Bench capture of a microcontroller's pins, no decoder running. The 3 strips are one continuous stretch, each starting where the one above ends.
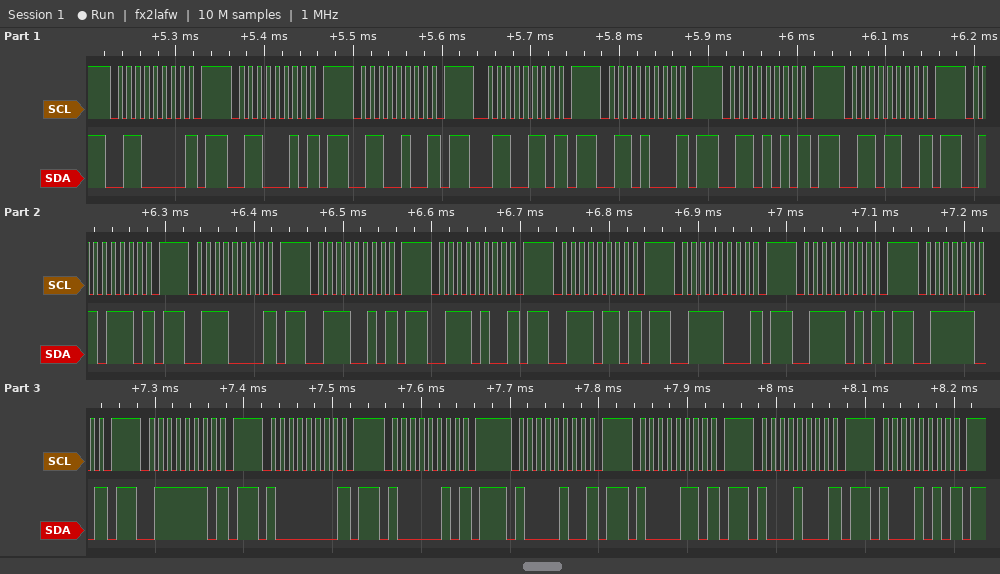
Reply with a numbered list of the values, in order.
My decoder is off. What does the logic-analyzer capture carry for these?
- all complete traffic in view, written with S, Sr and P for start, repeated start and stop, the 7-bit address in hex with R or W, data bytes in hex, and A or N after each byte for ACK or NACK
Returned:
1. S 30W N P S 31W N P S 32W N P S 33W N P S 34W N P S 35W N P S 36W N P S 37W N P S 38W N P S 39W N P S 3AW N P S 3BW N P S 3CW N P S 3DW N P S 3EW N P S 3FW N P S 40W N P S 41W N P S 42W N P S 43W N P S 44W N P S 45W N P
